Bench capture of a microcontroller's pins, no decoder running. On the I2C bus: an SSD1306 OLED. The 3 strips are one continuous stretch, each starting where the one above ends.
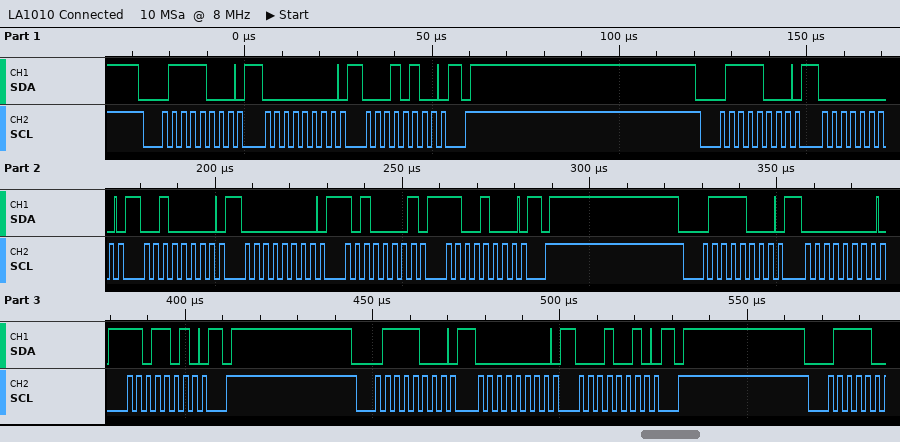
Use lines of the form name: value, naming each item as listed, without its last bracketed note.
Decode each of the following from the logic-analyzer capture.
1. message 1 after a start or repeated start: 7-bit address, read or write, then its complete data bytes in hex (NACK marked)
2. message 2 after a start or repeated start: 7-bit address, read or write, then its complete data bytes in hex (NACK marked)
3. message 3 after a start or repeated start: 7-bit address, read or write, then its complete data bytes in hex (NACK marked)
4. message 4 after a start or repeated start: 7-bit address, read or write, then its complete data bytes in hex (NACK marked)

message 1 after a start or repeated start: 7-bit address, read or write, then its complete data bytes in hex: 0x3C write: 00 14
message 2 after a start or repeated start: 7-bit address, read or write, then its complete data bytes in hex: 0x3C write: 00 20 00 A1 C8
message 3 after a start or repeated start: 7-bit address, read or write, then its complete data bytes in hex: 0x3C write: 00 DA
message 4 after a start or repeated start: 7-bit address, read or write, then its complete data bytes in hex: 0x3C write: 00 12
